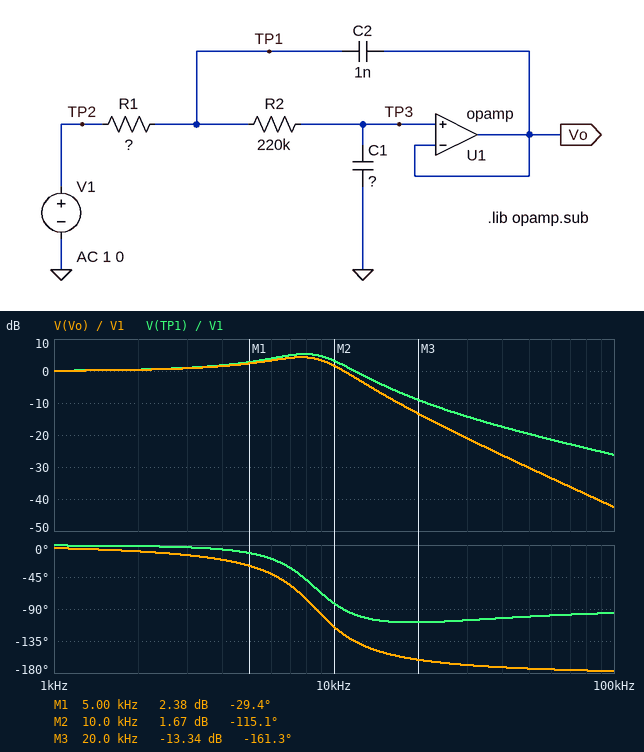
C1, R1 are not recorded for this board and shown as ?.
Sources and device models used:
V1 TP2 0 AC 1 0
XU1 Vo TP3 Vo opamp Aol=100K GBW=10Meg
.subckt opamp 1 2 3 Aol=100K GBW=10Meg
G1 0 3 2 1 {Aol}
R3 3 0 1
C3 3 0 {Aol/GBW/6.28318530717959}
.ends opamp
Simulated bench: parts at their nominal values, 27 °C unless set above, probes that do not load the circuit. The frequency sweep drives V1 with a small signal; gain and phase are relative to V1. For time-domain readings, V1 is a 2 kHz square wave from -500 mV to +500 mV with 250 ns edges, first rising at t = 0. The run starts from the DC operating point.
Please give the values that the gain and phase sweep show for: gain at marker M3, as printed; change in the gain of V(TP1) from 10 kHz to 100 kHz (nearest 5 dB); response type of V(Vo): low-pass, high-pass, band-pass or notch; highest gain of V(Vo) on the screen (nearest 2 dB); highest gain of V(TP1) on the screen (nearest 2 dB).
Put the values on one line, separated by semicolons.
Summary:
-13.34 dB; -30 dB; low-pass; 4 dB; 6 dB
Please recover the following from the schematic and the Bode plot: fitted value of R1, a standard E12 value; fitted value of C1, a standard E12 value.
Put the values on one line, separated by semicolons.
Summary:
33 kΩ; 47 pF
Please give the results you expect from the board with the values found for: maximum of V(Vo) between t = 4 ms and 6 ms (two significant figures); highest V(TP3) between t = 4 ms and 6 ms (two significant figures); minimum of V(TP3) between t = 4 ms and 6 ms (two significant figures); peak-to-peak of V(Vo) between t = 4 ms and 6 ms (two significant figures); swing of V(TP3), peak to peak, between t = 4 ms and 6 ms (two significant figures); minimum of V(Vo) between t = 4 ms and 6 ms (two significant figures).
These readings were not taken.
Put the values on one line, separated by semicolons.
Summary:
840 mV; 840 mV; -840 mV; 1.7 V; 1.7 V; -840 mV
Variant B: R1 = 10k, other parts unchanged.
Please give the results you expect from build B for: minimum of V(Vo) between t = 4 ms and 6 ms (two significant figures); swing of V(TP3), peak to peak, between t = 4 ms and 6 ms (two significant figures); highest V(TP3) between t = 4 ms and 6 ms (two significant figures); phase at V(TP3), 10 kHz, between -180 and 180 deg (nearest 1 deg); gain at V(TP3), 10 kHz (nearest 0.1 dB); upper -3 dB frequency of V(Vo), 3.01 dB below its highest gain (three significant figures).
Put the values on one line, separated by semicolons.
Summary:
-640 mV; 1.3 V; 640 mV; -49 deg; 0.9 dB; 18.1 kHz
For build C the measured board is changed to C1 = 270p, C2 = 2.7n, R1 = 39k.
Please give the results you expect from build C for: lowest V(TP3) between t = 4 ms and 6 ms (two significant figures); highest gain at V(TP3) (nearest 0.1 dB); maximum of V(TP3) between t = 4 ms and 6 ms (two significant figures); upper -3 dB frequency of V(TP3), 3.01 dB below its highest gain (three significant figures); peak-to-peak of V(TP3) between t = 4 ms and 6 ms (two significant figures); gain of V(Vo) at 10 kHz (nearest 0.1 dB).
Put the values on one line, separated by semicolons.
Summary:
-740 mV; 2.0 dB; 740 mV; 2.38 kHz; 1.5 V; -27.6 dB
